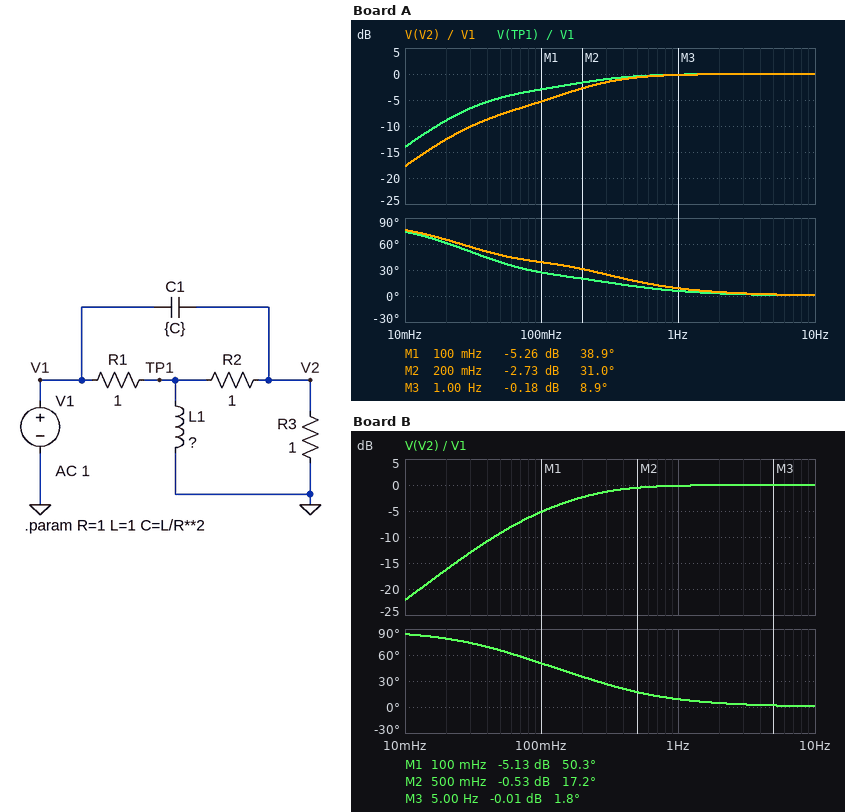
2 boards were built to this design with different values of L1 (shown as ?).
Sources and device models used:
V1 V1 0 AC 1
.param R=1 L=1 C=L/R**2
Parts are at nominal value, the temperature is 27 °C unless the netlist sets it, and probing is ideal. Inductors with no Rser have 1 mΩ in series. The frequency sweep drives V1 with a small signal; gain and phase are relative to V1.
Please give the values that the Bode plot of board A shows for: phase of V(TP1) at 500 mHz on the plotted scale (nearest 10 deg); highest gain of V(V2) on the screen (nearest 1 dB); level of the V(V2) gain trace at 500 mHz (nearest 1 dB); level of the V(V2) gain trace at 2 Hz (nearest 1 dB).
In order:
10 deg
0 dB
-1 dB
0 dB
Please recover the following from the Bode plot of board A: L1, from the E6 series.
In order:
3.3 H
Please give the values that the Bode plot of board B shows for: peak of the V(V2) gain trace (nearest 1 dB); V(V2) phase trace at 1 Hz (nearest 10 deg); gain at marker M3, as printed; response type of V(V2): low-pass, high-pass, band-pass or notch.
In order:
0 dB
10 deg
-0.01 dB
high-pass
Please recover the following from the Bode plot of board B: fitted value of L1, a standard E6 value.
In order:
1.5 H
